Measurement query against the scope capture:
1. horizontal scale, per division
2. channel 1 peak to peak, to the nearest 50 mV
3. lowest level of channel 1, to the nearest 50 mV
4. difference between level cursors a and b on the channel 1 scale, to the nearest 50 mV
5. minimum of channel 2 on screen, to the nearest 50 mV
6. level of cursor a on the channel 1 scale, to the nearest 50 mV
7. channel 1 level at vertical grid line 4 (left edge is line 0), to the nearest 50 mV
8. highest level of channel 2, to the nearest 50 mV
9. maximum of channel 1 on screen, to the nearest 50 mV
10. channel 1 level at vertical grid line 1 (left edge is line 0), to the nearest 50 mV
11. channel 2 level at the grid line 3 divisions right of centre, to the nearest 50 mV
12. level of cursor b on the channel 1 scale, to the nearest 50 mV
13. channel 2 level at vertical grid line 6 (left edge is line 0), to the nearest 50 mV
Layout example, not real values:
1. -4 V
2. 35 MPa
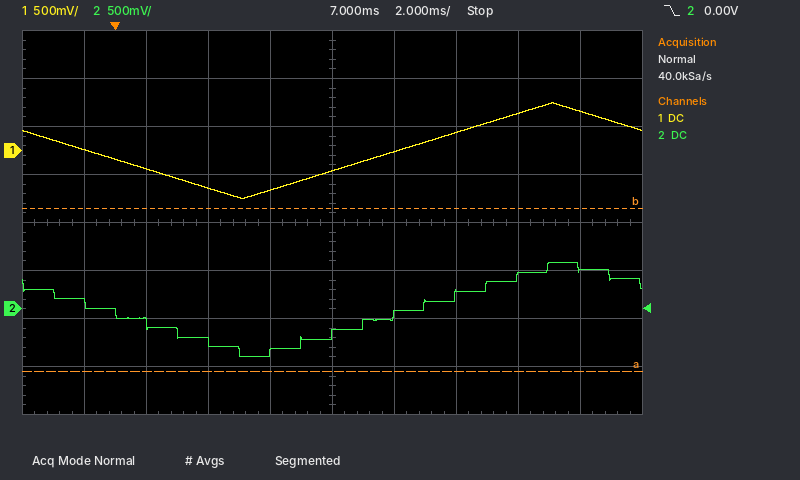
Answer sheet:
1. 2 ms
2. 1.00 V
3. -500 mV
4. 1.70 V
5. -500 mV
6. -2.30 V
7. -400 mV
8. 500 mV
9. 500 mV
10. 0 mV
11. 350 mV
12. -600 mV
13. -50 mV
